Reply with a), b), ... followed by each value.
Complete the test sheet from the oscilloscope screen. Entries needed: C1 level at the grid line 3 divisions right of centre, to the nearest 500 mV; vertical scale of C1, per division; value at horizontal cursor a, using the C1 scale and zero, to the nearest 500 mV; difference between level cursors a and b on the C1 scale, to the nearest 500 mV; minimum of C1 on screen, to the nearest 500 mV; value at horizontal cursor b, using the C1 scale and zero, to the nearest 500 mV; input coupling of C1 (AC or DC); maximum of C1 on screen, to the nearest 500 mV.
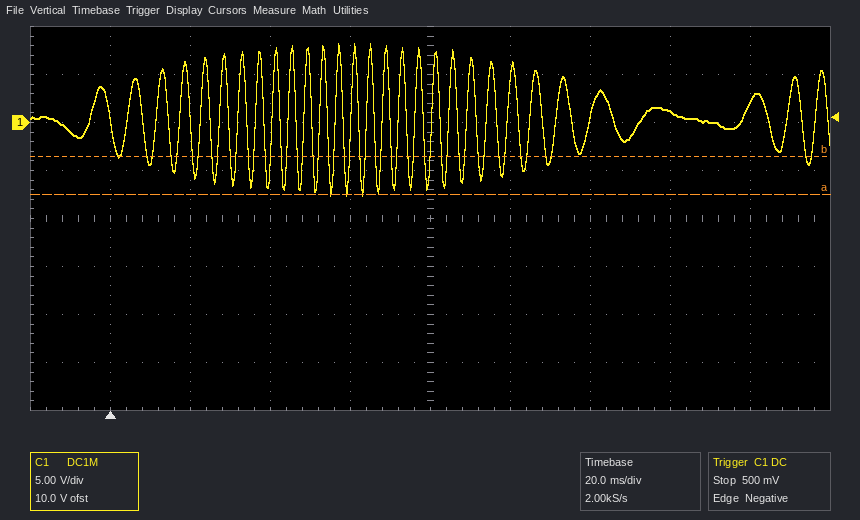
a) 1.0 V
b) 5 V
c) -7.5 V
d) 4.0 V
e) -7.5 V
f) -3.5 V
g) DC
h) 8.0 V
